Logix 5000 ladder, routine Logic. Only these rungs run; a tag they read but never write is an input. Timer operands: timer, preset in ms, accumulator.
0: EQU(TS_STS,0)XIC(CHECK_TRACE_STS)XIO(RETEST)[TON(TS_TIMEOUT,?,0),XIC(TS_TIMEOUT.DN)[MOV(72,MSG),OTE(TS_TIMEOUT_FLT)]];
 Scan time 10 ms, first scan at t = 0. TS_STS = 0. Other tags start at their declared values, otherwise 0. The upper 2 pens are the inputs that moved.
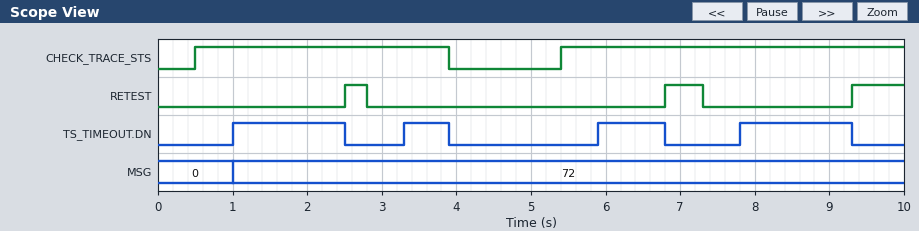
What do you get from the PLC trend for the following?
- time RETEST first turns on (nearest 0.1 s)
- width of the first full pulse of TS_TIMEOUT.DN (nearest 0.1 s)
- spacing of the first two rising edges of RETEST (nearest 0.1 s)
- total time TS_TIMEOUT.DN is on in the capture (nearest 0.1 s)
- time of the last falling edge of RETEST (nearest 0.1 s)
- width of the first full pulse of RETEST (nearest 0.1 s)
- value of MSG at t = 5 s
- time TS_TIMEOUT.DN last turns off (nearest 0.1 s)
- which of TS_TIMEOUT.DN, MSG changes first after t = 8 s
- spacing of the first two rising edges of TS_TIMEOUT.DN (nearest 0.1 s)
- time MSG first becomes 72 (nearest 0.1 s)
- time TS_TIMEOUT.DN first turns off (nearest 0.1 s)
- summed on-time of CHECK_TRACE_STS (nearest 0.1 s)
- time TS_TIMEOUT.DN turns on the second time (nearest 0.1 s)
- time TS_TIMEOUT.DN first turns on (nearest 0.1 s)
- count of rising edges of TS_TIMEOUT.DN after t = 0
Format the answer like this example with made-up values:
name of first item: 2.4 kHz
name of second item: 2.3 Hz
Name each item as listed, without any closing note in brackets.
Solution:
time RETEST first turns on: 2.5 s
width of the first full pulse of TS_TIMEOUT.DN: 1.5 s
spacing of the first two rising edges of RETEST: 4.3 s
total time TS_TIMEOUT.DN is on in the capture: 4.5 s
time of the last falling edge of RETEST: 7.3 s
width of the first full pulse of RETEST: 0.3 s
value of MSG at t = 5 s: 72
time TS_TIMEOUT.DN last turns off: 9.3 s
which of TS_TIMEOUT.DN, MSG changes first after t = 8 s: TS_TIMEOUT.DN
spacing of the first two rising edges of TS_TIMEOUT.DN: 2.3 s
time MSG first becomes 72: 1.0 s
time TS_TIMEOUT.DN first turns off: 2.5 s
summed on-time of CHECK_TRACE_STS: 8.0 s
time TS_TIMEOUT.DN turns on the second time: 3.3 s
time TS_TIMEOUT.DN first turns on: 1.0 s
count of rising edges of TS_TIMEOUT.DN after t = 0: 4
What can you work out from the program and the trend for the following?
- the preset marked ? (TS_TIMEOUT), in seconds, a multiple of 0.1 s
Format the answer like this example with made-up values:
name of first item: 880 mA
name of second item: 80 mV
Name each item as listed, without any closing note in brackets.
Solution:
the preset marked ? (TS_TIMEOUT), in seconds, a multiple of 0.1 s: 0.5 s
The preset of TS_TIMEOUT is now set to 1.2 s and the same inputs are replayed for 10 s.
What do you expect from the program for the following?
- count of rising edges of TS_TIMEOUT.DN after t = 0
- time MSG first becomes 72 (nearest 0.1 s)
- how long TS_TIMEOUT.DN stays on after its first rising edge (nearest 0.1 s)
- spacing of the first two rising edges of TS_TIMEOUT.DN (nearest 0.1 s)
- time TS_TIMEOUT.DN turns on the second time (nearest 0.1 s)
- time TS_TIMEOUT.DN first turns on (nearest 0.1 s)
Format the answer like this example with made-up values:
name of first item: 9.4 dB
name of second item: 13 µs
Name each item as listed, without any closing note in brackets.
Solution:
count of rising edges of TS_TIMEOUT.DN after t = 0: 3
time MSG first becomes 72: 1.7 s
how long TS_TIMEOUT.DN stays on after its first rising edge: 0.8 s
spacing of the first two rising edges of TS_TIMEOUT.DN: 4.9 s
time TS_TIMEOUT.DN turns on the second time: 6.6 s
time TS_TIMEOUT.DN first turns on: 1.7 s
